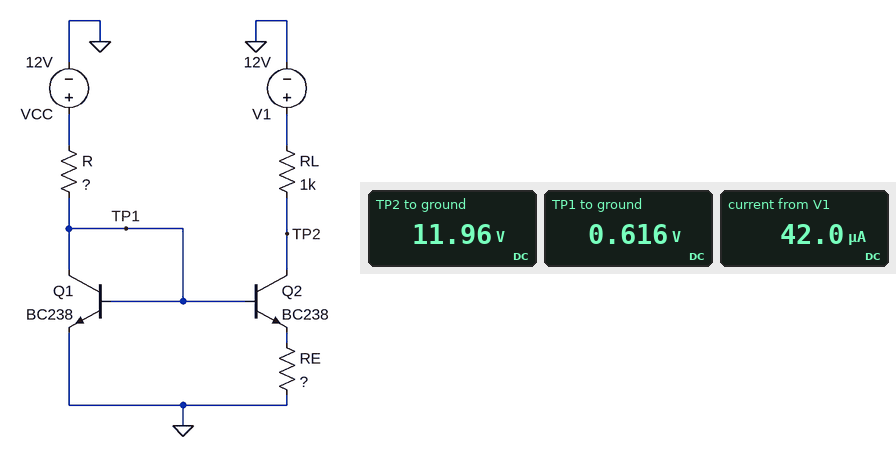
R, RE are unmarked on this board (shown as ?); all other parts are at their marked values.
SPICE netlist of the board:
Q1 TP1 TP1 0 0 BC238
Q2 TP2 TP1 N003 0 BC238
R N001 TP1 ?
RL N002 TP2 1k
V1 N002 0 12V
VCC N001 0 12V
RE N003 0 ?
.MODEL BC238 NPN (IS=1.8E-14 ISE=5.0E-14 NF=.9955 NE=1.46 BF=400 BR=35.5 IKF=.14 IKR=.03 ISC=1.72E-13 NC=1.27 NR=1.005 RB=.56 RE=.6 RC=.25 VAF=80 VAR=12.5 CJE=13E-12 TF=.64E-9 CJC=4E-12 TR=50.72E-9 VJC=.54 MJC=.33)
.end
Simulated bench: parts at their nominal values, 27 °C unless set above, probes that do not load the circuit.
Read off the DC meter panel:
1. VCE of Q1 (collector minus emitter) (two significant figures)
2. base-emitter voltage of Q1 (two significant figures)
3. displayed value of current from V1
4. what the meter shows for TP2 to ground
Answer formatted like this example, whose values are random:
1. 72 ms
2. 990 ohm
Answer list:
1. 620 mV
2. 620 mV
3. 42.0 µA
4. 11.96 V
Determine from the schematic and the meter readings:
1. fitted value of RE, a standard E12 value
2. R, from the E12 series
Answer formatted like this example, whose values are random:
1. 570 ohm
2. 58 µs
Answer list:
1. 1.5 kΩ
2. 27 kΩ
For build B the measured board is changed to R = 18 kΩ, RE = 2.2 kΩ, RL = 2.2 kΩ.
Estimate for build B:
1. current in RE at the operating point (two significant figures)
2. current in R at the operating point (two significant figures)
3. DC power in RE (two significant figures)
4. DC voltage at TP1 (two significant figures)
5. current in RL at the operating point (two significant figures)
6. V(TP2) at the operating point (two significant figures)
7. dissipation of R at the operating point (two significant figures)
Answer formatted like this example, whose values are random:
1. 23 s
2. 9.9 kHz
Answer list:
1. 36 µA
2. 630 µA
3. 2.8 µW
4. 630 mV
5. 35 µA
6. 12 V
7. 7.2 mW
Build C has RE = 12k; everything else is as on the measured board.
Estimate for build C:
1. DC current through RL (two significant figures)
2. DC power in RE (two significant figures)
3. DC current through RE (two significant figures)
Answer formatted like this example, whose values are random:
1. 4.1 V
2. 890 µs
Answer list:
1. 8.6 µA
2. 900 nW
3. 8.7 µA
